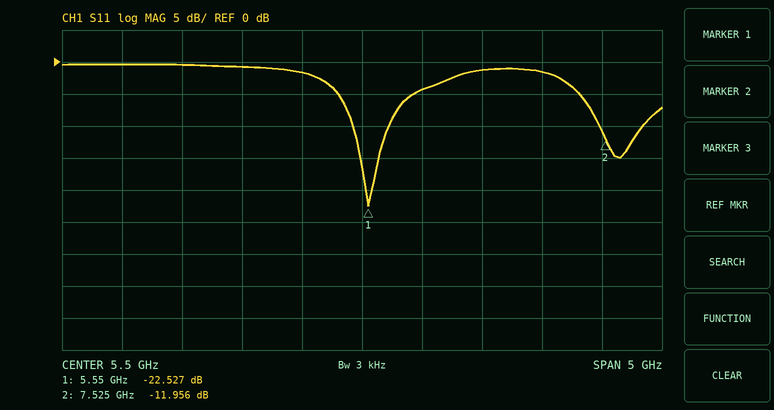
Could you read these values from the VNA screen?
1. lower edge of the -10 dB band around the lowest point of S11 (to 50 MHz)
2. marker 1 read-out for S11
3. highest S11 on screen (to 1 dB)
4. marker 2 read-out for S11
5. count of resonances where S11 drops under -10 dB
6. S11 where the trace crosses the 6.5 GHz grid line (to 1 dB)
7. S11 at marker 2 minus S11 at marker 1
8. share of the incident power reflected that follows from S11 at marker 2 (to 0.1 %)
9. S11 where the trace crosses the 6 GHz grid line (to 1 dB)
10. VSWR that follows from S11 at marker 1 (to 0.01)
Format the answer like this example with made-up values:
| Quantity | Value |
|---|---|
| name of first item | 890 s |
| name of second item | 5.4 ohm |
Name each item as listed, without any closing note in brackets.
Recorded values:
| Quantity | Value |
|---|---|
| lower edge of the -10 dB band around the lowest point of S11 | 5.40 GHz |
| marker 1 read-out for S11 | -22.527 dB |
| highest S11 on screen | 0 dB |
| marker 2 read-out for S11 | -11.956 dB |
| count of resonances where S11 drops under -10 dB | 2 |
| S11 where the trace crosses the 6.5 GHz grid line | -1 dB |
| S11 at marker 2 minus S11 at marker 1 | 10.571 dB |
| share of the incident power reflected that follows from S11 at marker 2 | 6.4 % |
| S11 where the trace crosses the 6 GHz grid line | -4 dB |
| VSWR that follows from S11 at marker 1 | 1.16 |
